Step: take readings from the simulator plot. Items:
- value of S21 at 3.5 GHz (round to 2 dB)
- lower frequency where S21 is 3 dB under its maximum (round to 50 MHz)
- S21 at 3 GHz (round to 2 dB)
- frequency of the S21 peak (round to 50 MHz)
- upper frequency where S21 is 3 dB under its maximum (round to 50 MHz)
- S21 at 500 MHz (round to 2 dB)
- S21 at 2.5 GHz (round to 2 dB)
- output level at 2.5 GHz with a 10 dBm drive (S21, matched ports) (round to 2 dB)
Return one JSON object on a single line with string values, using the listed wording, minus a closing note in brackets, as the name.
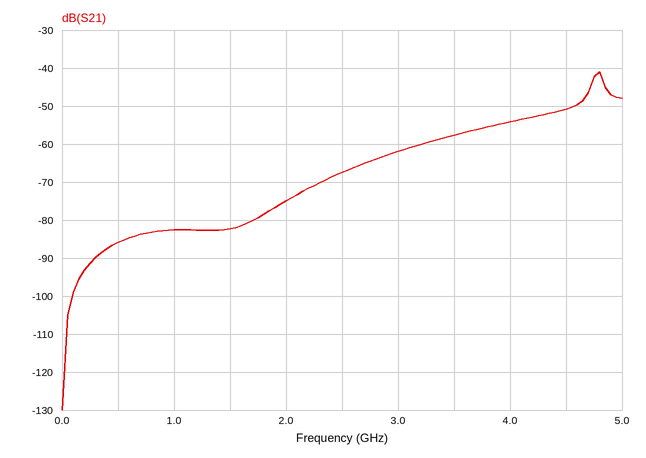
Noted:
{"value of S21 at 3.5 GHz": "-58 dB", "lower frequency where S21 is 3 dB under its maximum": "4.75 GHz", "S21 at 3 GHz": "-62 dB", "frequency of the S21 peak": "4.80 GHz", "upper frequency where S21 is 3 dB under its maximum": "4.85 GHz", "S21 at 500 MHz": "-86 dB", "S21 at 2.5 GHz": "-68 dB", "output level at 2.5 GHz with a 10 dBm drive (S21, matched ports)": "-58 dBm"}
